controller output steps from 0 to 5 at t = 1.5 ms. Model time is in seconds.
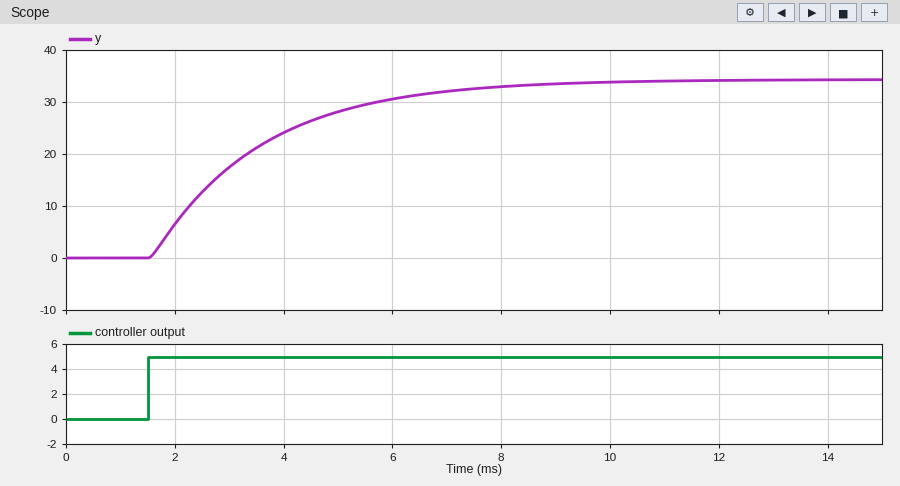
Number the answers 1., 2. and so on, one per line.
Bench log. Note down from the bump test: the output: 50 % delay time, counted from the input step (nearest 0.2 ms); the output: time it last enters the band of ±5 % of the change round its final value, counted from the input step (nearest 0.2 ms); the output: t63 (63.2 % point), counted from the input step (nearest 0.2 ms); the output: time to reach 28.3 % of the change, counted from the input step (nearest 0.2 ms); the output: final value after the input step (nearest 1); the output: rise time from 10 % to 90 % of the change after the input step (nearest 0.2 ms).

1. 1.4 ms
2. 6.0 ms
3. 2.0 ms
4. 0.8 ms
5. 34
6. 4.4 ms
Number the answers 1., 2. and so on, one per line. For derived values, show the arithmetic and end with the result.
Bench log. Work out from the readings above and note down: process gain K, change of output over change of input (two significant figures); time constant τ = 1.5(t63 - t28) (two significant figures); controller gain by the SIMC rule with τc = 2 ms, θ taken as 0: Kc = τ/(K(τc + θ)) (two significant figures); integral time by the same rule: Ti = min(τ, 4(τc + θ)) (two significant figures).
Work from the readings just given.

1. (34 - 0) / 5 = 6.8
2. 1.5 × (2 - 0.8) = 1.8 ms
3. 1.8 / (6.8 × (2 + 0)) = 0.13
4. min(1.8, 4 × (2 + 0)) = 1.8 ms
